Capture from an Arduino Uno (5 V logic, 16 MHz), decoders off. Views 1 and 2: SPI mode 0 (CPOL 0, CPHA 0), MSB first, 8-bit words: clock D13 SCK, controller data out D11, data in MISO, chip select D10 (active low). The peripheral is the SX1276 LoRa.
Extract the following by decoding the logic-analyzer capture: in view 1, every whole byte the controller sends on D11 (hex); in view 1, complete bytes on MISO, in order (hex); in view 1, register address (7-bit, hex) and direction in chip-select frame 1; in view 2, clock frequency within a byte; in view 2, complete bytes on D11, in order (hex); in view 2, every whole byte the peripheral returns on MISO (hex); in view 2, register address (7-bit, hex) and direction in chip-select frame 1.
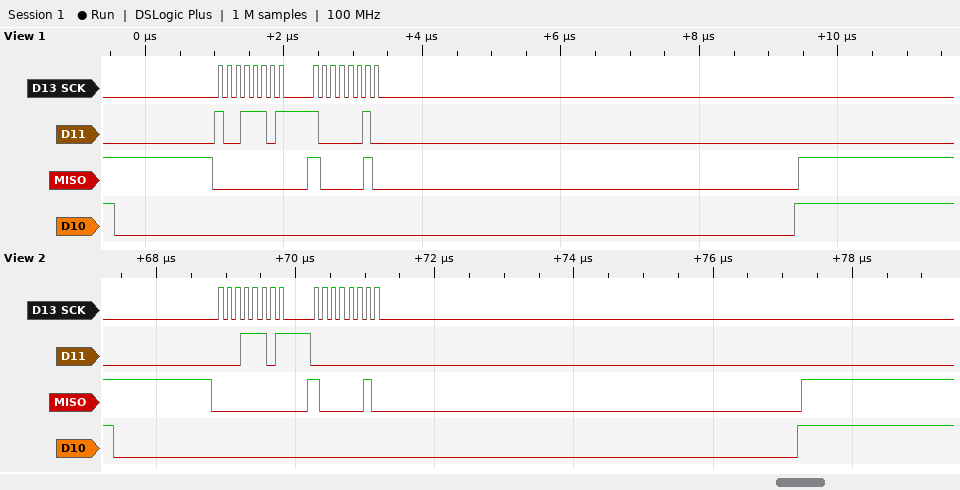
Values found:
0x9D 0x82
0x00 0x82
0x1D write
8 MHz
1D 00
00 82
0x1D read
